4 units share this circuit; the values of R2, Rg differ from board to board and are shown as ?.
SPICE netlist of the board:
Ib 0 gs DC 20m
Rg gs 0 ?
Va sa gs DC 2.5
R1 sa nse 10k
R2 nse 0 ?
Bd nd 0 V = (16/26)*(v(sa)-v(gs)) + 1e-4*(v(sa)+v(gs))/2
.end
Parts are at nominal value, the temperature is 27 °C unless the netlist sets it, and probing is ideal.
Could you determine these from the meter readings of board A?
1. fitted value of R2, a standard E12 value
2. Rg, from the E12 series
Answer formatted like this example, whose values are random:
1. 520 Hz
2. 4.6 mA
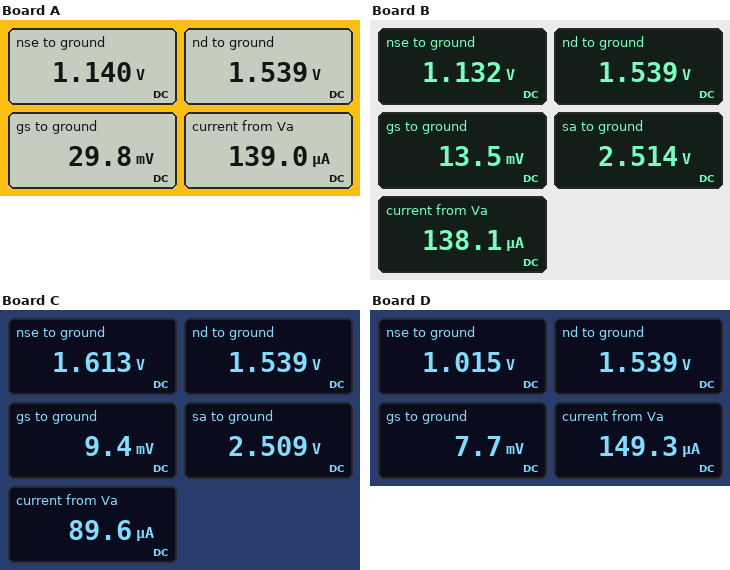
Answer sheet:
1. 8.2 kΩ
2. 1.5 Ω
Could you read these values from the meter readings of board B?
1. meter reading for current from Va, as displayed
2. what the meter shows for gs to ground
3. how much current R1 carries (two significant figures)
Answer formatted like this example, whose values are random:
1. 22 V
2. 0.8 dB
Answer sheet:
1. 138.1 µA
2. 13.5 mV
3. 140 µA
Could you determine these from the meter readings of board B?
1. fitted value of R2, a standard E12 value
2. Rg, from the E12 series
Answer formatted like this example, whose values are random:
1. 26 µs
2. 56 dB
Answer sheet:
1. 8.2 kΩ
2. 0.68 Ω
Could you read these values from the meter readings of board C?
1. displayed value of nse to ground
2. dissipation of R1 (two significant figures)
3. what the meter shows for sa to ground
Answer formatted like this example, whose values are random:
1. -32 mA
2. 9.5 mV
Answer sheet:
1. 1.613 V
2. 80 µW
3. 2.509 V
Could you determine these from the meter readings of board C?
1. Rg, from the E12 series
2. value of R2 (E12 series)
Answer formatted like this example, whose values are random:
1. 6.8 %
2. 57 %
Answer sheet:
1. 0.47 Ω
2. 18 kΩ
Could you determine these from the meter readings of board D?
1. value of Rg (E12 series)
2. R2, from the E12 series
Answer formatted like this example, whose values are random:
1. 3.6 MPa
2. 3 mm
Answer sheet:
1. 0.39 Ω
2. 6.8 kΩ
